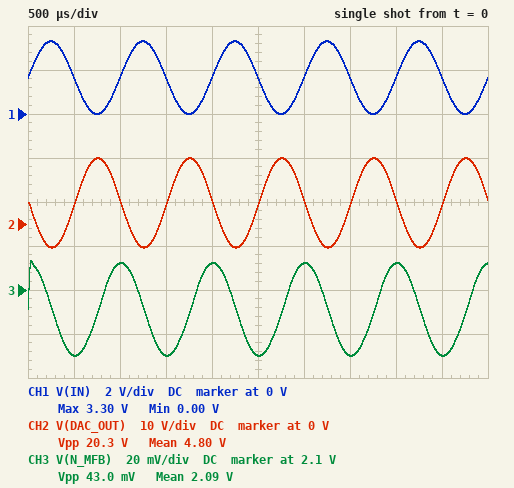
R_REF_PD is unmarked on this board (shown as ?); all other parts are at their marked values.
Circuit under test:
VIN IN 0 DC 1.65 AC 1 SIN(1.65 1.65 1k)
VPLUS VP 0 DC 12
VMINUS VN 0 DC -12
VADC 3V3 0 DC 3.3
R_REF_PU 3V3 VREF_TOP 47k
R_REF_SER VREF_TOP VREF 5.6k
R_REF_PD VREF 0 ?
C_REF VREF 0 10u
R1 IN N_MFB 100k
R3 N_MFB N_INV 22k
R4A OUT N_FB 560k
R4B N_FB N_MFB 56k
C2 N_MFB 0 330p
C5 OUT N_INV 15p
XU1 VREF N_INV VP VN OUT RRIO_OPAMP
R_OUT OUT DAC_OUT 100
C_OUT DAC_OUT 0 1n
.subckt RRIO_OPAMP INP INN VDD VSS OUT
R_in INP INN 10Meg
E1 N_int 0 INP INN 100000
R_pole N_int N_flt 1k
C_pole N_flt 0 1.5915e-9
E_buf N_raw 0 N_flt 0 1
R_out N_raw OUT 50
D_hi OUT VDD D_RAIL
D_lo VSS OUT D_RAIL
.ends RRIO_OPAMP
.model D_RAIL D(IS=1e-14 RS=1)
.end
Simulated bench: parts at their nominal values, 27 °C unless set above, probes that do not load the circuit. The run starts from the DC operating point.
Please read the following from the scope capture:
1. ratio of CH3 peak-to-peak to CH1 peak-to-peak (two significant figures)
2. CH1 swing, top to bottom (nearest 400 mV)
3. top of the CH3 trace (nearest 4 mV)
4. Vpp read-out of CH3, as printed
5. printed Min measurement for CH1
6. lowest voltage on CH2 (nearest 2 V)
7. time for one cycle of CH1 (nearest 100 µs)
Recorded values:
0.013
3.2 V
2.112 V
43.0 mV
0.00 V
-6 V
1.0 ms
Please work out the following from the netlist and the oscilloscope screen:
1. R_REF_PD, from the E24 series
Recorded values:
91 kΩ
